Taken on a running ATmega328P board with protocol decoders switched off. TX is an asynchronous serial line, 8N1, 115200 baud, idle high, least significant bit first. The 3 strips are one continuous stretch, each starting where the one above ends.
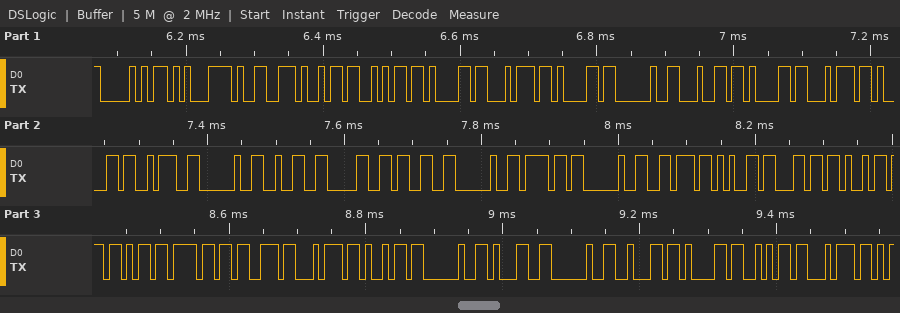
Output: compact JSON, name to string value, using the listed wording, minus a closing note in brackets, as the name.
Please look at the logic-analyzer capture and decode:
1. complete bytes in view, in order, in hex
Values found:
{"complete bytes in view, in order, in hex": "50 C5 99 69 6A 61 74 61 20 64 61 74 61 3A 20 32 30 33 20 6F 20 76 65 6C 69 6B 6F 73 74 69 20 31 20 62 61 6A 74"}
